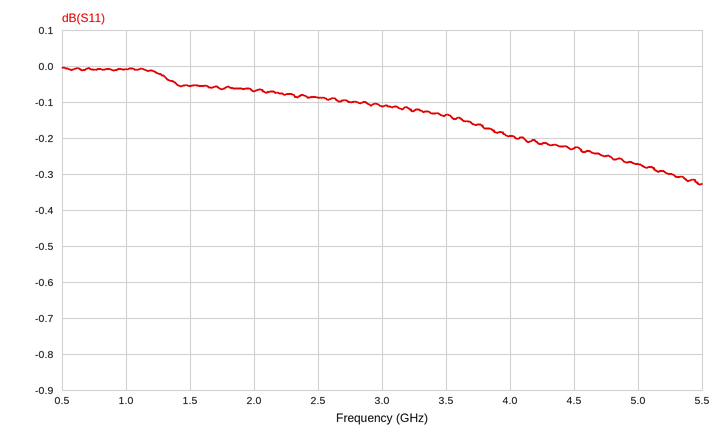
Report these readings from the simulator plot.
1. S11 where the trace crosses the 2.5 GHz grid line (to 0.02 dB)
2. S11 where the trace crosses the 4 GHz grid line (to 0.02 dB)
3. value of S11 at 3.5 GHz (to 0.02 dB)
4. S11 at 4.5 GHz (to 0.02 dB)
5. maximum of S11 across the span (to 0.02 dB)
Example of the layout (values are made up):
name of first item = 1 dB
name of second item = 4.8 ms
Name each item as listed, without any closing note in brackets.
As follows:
S11 where the trace crosses the 2.5 GHz grid line = -0.08 dB
S11 where the trace crosses the 4 GHz grid line = -0.20 dB
value of S11 at 3.5 GHz = -0.14 dB
S11 at 4.5 GHz = -0.22 dB
maximum of S11 across the span = 0.00 dB
